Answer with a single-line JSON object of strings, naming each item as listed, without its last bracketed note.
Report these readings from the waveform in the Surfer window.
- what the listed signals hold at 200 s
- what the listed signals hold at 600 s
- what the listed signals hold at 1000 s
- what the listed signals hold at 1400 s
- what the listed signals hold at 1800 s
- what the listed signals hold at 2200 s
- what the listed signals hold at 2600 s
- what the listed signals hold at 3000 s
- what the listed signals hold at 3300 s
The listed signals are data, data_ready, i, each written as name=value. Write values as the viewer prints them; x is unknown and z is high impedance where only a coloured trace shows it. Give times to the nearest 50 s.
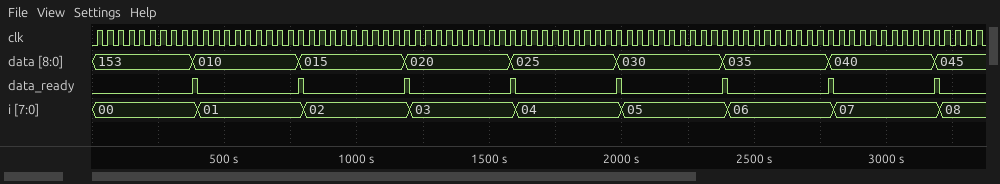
{"what the listed signals hold at 200 s": "data=153, data_ready=0, i=00", "what the listed signals hold at 600 s": "data=010, data_ready=0, i=01", "what the listed signals hold at 1000 s": "data=015, data_ready=0, i=02", "what the listed signals hold at 1400 s": "data=020, data_ready=0, i=03", "what the listed signals hold at 1800 s": "data=025, data_ready=0, i=04", "what the listed signals hold at 2200 s": "data=030, data_ready=0, i=05", "what the listed signals hold at 2600 s": "data=035, data_ready=0, i=06", "what the listed signals hold at 3000 s": "data=040, data_ready=0, i=07", "what the listed signals hold at 3300 s": "data=045, data_ready=0, i=08"}
